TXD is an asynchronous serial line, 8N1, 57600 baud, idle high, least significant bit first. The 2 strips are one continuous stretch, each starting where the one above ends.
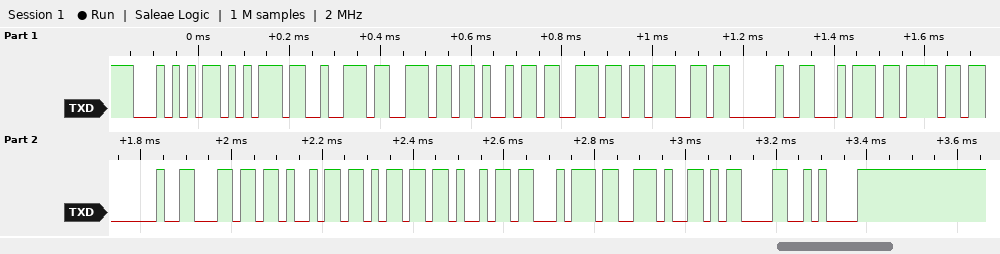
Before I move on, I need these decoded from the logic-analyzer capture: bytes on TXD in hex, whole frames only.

0x54 0x75 0x72 0x6E 0x69 0x6E 0x67 0x20 0x74 0x6F 0x20 0x6C 0x69 0x6D 0x69 0x74 0x2E 0x0D 0x0A
